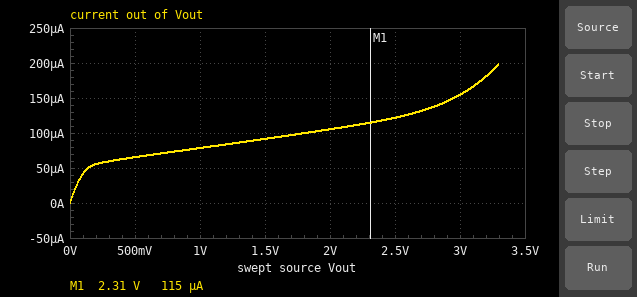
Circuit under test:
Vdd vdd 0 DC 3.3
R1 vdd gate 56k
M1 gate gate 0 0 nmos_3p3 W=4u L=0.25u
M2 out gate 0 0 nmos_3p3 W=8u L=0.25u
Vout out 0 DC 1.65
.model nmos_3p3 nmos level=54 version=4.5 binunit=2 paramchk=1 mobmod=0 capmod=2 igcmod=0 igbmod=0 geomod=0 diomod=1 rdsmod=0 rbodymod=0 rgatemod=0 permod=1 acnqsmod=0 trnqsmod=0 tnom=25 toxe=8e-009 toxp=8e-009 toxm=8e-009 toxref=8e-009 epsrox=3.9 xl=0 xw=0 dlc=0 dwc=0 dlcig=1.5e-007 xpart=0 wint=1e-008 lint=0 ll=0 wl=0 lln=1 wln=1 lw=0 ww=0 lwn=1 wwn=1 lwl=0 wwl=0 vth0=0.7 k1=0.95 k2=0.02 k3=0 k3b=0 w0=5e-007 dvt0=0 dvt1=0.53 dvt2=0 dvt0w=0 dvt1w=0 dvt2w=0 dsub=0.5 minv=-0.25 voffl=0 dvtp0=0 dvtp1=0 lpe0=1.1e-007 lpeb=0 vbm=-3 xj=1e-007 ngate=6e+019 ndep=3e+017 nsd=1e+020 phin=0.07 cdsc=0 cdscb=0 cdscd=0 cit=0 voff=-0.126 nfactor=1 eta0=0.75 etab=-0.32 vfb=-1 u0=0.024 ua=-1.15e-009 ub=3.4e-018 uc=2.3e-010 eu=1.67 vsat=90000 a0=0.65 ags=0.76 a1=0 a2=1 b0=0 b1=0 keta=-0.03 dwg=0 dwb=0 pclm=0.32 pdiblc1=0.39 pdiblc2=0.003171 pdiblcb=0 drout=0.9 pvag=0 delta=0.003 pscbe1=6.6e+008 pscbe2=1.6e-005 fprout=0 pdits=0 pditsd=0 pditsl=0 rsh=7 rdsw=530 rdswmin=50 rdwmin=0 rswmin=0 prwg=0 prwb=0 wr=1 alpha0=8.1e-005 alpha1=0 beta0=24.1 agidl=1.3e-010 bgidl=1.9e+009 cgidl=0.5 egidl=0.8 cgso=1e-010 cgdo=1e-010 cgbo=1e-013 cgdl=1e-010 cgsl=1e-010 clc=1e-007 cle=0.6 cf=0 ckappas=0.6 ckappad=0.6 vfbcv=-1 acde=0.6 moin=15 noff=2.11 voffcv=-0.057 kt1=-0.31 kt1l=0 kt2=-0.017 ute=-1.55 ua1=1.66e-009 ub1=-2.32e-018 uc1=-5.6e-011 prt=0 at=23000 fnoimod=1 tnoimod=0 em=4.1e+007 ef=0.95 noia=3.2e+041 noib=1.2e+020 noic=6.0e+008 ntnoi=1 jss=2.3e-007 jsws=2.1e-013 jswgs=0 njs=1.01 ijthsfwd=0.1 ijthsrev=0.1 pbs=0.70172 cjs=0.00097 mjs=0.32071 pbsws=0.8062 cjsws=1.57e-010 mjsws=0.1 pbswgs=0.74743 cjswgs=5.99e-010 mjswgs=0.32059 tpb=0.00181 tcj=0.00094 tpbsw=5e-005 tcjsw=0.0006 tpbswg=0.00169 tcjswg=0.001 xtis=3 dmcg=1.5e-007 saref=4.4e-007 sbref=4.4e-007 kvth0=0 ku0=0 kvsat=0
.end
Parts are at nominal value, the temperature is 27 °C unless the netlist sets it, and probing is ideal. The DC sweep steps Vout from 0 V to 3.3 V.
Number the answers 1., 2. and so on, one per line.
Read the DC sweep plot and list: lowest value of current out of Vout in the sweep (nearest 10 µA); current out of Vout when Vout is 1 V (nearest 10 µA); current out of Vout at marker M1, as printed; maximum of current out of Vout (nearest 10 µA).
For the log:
1. 0 A
2. 80 µA
3. 115 µA
4. 200 µA
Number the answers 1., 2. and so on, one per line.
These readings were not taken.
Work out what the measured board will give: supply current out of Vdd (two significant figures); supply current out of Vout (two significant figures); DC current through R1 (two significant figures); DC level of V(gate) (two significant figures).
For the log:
1. 40 µA
2. 96 µA
3. 40 µA
4. 1.1 V
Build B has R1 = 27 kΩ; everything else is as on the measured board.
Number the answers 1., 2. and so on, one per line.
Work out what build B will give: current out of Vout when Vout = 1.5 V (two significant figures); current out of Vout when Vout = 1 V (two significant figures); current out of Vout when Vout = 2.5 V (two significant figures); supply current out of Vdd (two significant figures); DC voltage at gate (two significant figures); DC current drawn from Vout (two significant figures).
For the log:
1. 170 µA
2. 150 µA
3. 210 µA
4. 79 µA
5. 1.2 V
6. 180 µA
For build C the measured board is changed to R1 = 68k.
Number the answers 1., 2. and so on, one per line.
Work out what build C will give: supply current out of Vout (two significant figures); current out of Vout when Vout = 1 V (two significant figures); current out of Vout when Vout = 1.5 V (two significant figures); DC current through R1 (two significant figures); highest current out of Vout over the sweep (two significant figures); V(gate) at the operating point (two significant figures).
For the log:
1. 81 µA
2. 66 µA
3. 78 µA
4. 33 µA
5. 180 µA
6. 1.0 V
